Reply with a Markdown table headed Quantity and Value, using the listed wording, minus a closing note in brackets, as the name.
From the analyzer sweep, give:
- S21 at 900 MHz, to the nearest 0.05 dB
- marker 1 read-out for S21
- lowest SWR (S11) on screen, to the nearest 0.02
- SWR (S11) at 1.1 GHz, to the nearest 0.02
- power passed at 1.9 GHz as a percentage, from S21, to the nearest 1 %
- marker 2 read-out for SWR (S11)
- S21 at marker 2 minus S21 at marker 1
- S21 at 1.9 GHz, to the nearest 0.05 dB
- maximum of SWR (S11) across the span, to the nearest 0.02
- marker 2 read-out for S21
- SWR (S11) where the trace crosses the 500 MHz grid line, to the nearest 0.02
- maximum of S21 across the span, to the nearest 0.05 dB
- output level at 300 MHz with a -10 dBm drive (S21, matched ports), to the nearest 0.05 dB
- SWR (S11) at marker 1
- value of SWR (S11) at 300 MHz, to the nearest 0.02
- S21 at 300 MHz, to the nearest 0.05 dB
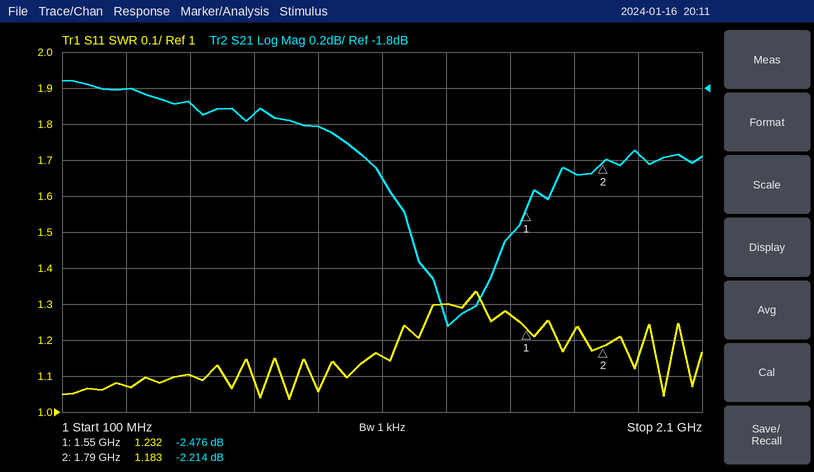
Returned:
| Quantity | Value |
|---|---|
| S21 at 900 MHz, to the nearest 0.05 dB | -2.00 dB |
| marker 1 read-out for S21 | -2.476 dB |
| lowest SWR (S11) on screen, to the nearest 0.02 | 1.04 |
| SWR (S11) at 1.1 GHz, to the nearest 0.02 | 1.16 |
| power passed at 1.9 GHz as a percentage, from S21, to the nearest 1 % | 61 % |
| marker 2 read-out for SWR | 1.183 |
| S21 at marker 2 minus S21 at marker 1 | 0.262 dB |
| S21 at 1.9 GHz, to the nearest 0.05 dB | -2.15 dB |
| maximum of SWR (S11) across the span, to the nearest 0.02 | 1.34 |
| marker 2 read-out for S21 | -2.214 dB |
| SWR (S11) where the trace crosses the 500 MHz grid line, to the nearest 0.02 | 1.10 |
| maximum of S21 across the span, to the nearest 0.05 dB | -1.75 dB |
| output level at 300 MHz with a -10 dBm drive (S21, matched ports), to the nearest 0.05 dB | -11.80 dBm |
| SWR (S11) at marker 1 | 1.232 |
| value of SWR (S11) at 300 MHz, to the nearest 0.02 | 1.08 |
| S21 at 300 MHz, to the nearest 0.05 dB | -1.80 dB |
